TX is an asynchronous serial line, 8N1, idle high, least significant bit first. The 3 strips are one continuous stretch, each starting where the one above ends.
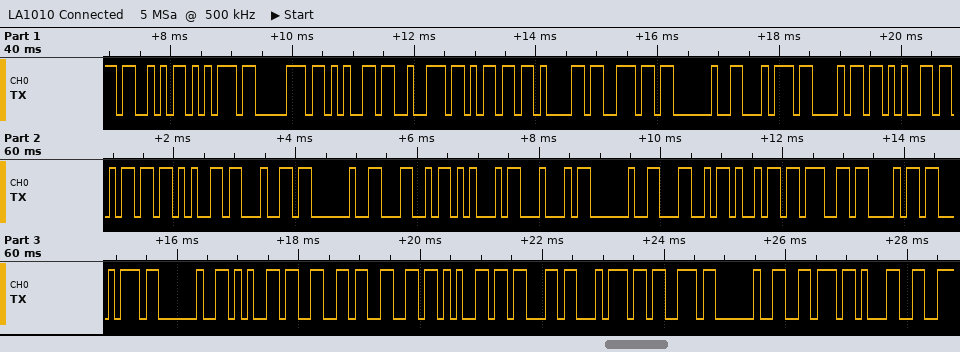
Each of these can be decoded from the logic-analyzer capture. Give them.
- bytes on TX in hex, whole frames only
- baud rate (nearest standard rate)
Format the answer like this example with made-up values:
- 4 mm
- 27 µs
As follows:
- 53 75 70 65 72 6D 61 6E 20 74 68 65 6D 65 64 20 4C 45 44 20 4C 69 67 68 74 20 65 66 66 65 63 74 73 20 76 31
- 9600 baud
